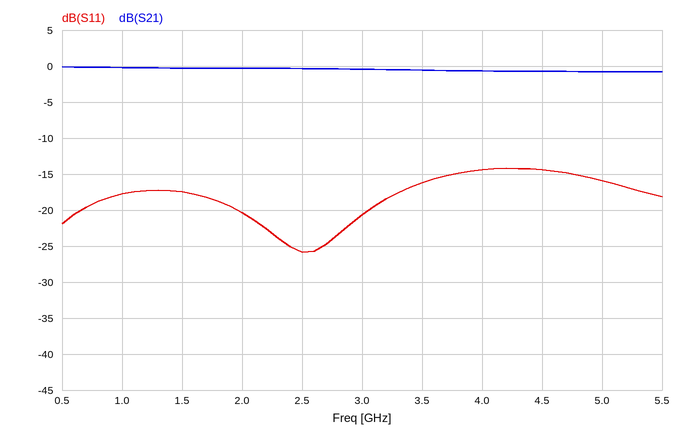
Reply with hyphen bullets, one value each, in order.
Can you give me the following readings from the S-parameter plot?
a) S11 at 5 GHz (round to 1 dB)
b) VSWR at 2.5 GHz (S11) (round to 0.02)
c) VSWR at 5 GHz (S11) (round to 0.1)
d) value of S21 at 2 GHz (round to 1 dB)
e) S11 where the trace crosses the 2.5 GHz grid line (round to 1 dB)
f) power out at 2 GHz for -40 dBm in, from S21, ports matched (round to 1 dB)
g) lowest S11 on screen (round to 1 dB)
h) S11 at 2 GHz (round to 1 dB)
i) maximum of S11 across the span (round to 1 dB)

- -16 dB
- 1.10
- 1.4
- 0 dB
- -26 dB
- -40 dBm
- -26 dB
- -20 dB
- -14 dB
